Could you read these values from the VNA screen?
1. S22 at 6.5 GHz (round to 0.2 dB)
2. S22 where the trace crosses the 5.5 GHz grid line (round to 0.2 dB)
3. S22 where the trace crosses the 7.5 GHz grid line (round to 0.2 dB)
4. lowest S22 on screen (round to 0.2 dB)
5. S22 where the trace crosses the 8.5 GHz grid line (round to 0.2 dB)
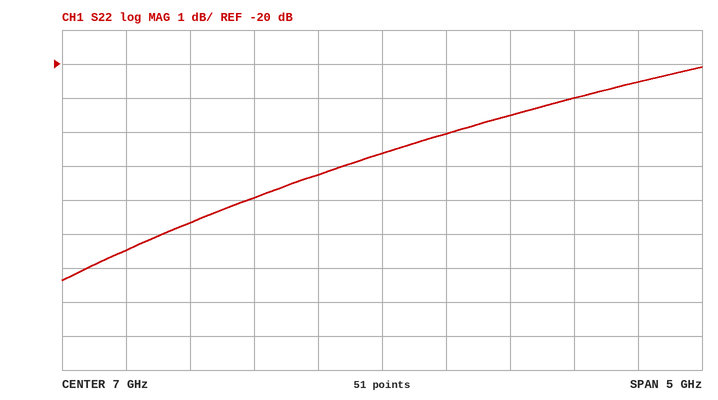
-23.2 dB
-24.6 dB
-22.0 dB
-26.4 dB
-21.0 dB
